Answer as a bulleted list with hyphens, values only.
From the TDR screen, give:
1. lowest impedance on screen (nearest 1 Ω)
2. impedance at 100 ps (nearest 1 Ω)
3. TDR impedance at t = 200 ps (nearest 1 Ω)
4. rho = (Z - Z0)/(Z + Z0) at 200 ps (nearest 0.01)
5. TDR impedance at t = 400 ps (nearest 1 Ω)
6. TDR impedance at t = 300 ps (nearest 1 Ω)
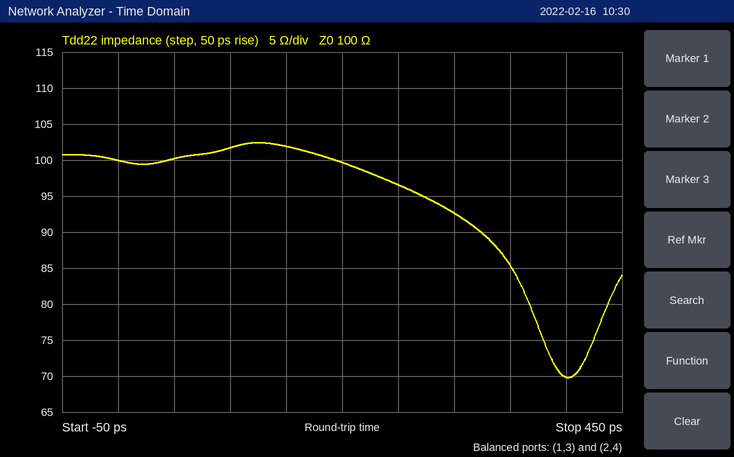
- 70 Ω
- 102 Ω
- 100 Ω
- 0.00
- 70 Ω
- 93 Ω
